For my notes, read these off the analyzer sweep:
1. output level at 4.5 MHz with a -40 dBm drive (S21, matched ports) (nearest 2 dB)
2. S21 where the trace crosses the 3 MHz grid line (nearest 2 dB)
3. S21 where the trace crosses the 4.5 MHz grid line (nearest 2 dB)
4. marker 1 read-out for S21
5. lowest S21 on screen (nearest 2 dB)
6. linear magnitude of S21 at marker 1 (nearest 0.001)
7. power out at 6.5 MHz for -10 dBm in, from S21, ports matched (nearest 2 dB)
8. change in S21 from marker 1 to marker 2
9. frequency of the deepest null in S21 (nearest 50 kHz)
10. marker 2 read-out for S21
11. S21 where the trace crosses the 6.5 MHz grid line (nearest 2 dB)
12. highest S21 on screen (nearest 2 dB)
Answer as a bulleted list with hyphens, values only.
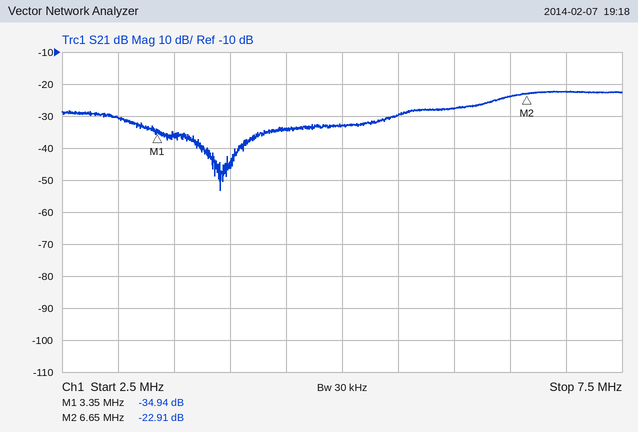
- -74 dBm
- -30 dB
- -34 dB
- -34.94 dB
- -54 dB
- 0.018
- -34 dBm
- 12.03 dB
- 3.90 MHz
- -22.91 dB
- -24 dB
- -22 dB
